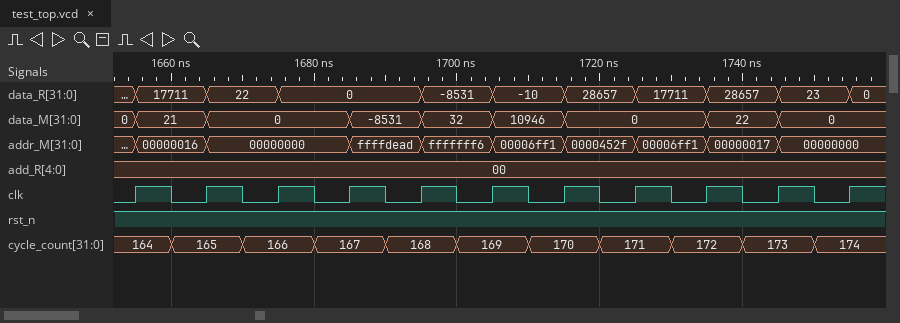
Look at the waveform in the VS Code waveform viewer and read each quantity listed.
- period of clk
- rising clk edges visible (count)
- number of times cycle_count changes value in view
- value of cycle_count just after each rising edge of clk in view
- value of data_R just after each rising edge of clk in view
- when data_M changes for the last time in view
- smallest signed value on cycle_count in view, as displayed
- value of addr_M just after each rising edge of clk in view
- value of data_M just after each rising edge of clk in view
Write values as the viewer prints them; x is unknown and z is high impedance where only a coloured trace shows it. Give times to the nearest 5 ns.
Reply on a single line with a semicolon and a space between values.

10 ns; 11; 10; 164, 165, 166, 167, 168, 169, 170, 171, 172, 173, 174; 17711, 22, 0, 0, -8531, -10, 28657, 17711, 28657, 23, 0; 1745 ns; 164; 00000016, 00000000, 00000000, ffffdead, fffffff6, 00006ff1, 0000452f, 00006ff1, 00000017, 00000000, 00000000; 21, 0, 0, -8531, 32, 10946, 0, 0, 22, 0, 0
